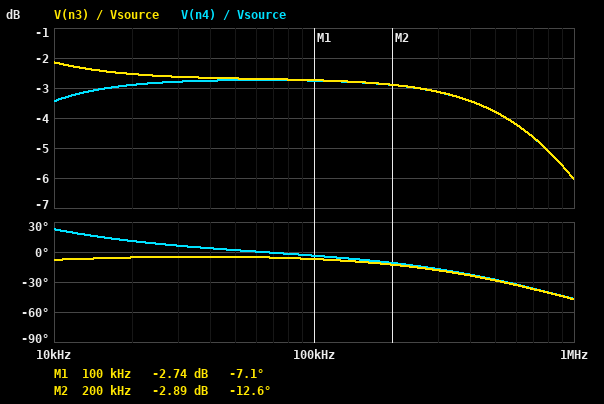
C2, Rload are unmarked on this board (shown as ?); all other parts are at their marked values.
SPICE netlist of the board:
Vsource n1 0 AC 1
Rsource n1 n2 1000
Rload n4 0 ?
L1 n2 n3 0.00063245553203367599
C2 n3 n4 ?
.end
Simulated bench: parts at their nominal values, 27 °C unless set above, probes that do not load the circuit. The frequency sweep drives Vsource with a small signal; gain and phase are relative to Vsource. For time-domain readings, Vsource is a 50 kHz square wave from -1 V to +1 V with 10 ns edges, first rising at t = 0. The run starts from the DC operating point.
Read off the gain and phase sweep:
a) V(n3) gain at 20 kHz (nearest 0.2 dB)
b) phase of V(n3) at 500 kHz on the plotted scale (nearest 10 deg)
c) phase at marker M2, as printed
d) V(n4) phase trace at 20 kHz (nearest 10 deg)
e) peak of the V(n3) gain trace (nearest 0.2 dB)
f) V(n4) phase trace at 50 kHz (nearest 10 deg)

-2.6 dB
-30 deg
-12.6 deg
10 deg
-2.2 dB
0 deg
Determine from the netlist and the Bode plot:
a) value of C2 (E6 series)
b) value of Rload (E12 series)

10 nF
2.7 kΩ
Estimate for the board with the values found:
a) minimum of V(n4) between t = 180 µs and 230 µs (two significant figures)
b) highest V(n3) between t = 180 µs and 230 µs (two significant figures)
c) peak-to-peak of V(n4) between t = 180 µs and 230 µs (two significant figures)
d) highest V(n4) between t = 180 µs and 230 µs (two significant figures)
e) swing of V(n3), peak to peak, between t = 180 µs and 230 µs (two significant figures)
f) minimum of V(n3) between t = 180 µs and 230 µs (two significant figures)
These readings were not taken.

-810 mV
770 mV
1.6 V
810 mV
1.5 V
-770 mV
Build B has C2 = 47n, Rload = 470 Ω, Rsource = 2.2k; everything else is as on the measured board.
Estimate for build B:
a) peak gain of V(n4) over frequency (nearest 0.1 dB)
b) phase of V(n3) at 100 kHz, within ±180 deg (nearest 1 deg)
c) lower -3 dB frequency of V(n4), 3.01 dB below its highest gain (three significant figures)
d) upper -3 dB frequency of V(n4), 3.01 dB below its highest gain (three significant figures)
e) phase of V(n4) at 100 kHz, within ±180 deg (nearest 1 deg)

-15.1 dB
-12 deg
1.27 kHz
673 kHz
-8 deg
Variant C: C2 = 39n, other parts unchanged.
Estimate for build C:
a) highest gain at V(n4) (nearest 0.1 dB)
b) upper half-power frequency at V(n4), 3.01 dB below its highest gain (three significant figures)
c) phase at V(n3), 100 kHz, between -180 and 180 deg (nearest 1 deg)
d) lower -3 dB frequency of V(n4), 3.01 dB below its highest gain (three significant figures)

-2.7 dB
932 kHz
-6 deg
1.10 kHz
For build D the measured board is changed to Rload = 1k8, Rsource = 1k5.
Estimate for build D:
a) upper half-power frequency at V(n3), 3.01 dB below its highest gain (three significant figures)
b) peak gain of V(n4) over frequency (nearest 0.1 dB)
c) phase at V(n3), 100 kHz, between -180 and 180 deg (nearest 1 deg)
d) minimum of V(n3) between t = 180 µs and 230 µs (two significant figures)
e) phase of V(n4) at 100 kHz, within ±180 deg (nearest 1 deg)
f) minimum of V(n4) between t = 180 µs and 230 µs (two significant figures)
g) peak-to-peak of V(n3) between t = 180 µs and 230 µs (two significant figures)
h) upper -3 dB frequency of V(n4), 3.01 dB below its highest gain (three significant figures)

7.69 kHz
-5.3 dB
-9 deg
-620 mV
-4 deg
-610 mV
1.2 V
835 kHz
